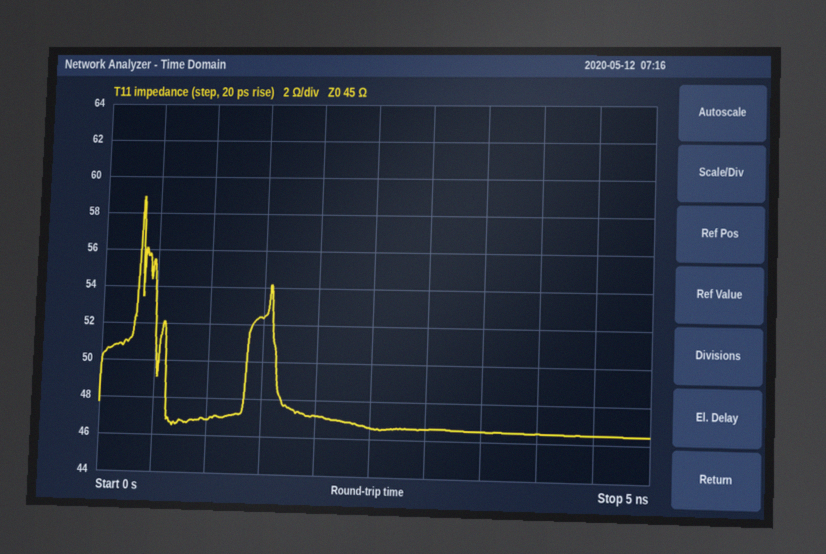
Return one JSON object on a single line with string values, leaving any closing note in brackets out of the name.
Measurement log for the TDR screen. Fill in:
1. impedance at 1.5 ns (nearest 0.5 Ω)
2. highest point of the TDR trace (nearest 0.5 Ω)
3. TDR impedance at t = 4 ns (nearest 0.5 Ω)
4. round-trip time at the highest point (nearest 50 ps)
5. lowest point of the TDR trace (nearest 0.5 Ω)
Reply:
{"impedance at 1.5 ns": "52.5 Ω", "highest point of the TDR trace": "59.0 Ω", "TDR impedance at t = 4 ns": "46.5 Ω", "round-trip time at the highest point": "350 ps", "lowest point of the TDR trace": "46.5 Ω"}
